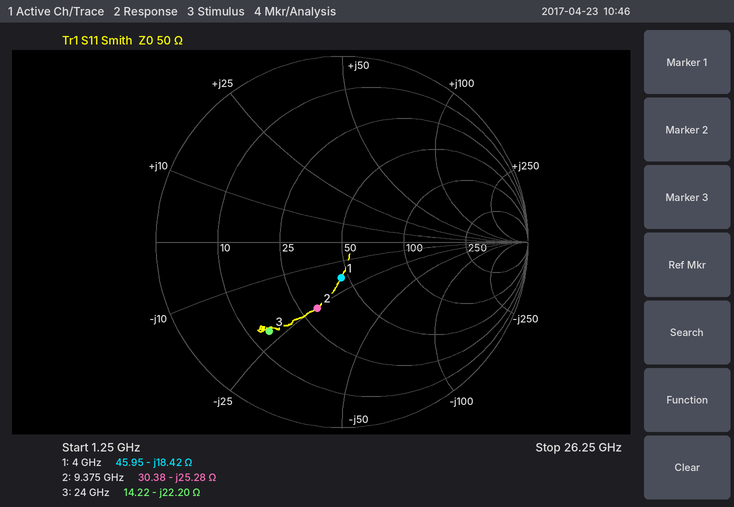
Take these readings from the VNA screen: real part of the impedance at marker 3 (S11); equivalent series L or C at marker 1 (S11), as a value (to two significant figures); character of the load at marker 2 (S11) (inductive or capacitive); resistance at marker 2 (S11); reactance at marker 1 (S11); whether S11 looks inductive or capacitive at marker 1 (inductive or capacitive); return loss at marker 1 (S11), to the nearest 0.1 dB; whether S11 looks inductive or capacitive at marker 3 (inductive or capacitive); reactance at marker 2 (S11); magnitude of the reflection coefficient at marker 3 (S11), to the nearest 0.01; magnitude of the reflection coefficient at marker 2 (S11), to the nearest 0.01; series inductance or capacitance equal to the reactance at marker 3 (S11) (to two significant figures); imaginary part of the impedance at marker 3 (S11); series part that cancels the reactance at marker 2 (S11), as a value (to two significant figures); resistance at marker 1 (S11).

14.22 Ω
2.2 pF
capacitive
30.38 Ω
-18.42 Ω
capacitive
14.3 dB
capacitive
-25.28 Ω
0.62
0.38
300 fF
-22.20 Ω
430 pH
45.95 Ω
